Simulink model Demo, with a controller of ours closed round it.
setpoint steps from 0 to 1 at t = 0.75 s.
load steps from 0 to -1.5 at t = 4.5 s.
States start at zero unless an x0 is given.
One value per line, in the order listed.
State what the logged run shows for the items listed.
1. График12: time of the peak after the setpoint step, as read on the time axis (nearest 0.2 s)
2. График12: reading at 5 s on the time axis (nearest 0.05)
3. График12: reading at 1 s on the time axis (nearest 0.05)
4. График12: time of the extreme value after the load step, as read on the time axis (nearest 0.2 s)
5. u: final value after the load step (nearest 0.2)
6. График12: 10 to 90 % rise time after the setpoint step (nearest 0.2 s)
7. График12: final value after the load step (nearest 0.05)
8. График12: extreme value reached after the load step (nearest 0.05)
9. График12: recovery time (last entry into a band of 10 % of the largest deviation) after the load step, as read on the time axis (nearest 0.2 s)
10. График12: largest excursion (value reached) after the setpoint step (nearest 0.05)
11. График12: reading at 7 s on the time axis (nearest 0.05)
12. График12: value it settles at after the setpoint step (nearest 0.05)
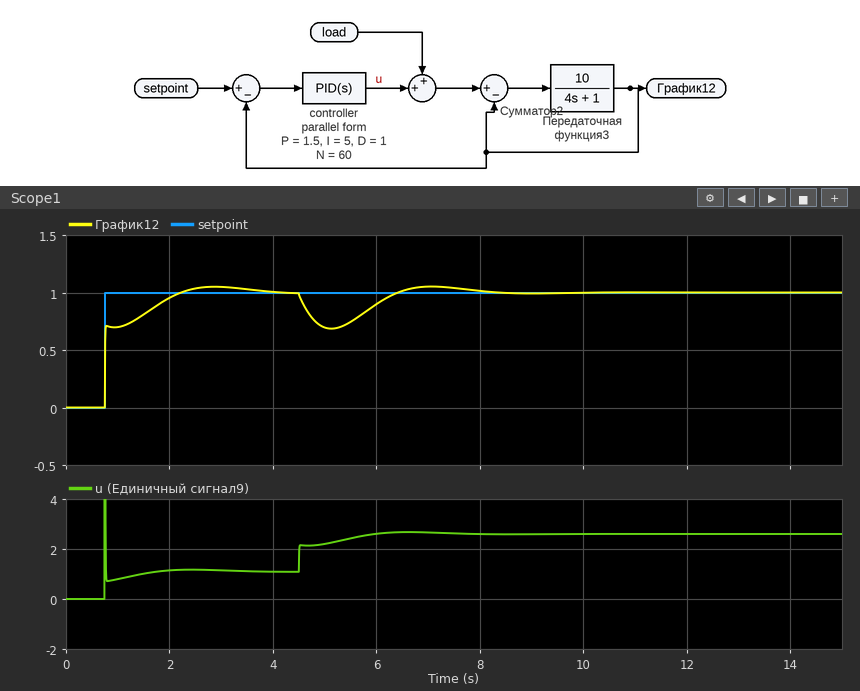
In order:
2.8 s
0.70
0.70
5.2 s
2.6
1.0 s
1.00
0.70
7.6 s
1.05
1.05
1.00
